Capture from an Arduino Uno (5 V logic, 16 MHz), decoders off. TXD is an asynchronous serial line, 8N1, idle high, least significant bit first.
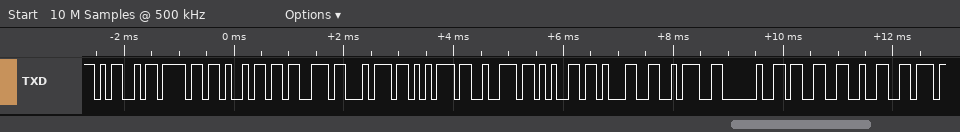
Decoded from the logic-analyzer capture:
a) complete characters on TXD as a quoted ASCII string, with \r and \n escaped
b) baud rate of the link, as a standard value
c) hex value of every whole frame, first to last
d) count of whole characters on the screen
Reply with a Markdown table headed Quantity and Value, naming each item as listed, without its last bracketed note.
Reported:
| Quantity | Value |
|---|---|
| complete characters on TXD as a quoted ASCII string, with \r and \n escaped | "Moisture1: 32" |
| baud rate of the link, as a standard value | 9600 baud |
| hex value of every whole frame, first to last | 4D 6F 69 73 74 75 72 65 31 3A 20 33 32 |
| count of whole characters on the screen | 13 |
